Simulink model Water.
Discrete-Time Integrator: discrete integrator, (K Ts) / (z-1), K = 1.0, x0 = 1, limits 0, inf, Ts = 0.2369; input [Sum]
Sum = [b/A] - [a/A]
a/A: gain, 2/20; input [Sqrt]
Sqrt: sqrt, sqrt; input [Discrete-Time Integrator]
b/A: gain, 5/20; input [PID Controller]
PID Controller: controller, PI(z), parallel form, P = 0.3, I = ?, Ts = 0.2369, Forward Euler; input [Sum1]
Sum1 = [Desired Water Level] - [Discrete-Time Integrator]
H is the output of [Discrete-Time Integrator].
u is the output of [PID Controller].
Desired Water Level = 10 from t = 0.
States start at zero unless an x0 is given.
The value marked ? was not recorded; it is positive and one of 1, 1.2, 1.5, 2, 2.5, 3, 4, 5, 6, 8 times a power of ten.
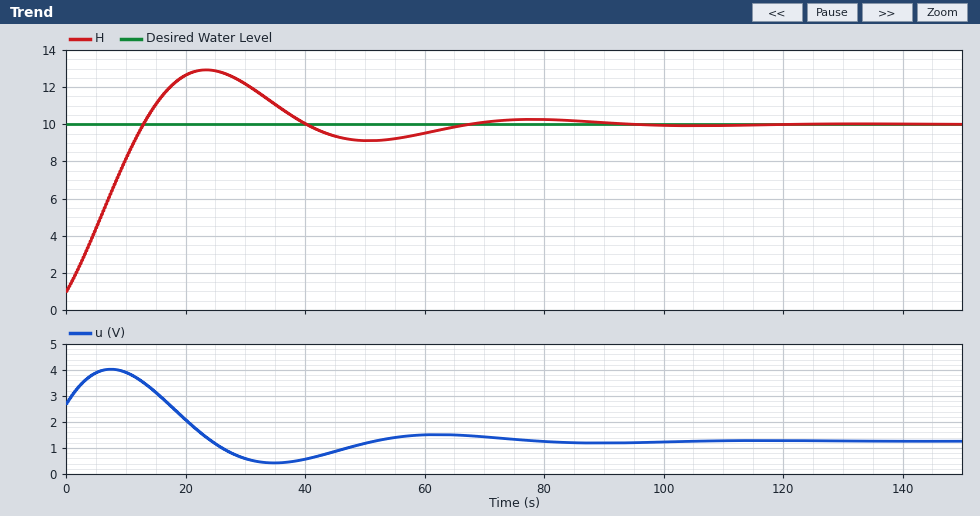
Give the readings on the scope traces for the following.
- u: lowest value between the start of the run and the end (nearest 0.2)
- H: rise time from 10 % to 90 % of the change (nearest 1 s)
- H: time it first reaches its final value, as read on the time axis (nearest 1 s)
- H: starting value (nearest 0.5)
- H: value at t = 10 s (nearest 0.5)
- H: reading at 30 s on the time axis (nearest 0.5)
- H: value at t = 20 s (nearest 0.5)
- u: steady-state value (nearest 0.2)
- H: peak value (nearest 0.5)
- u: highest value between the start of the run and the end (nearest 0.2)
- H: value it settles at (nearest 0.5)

0.4
10 s
13 s
1.0
8.0
12.0
12.5
1.2
13.0
4.0
10.0
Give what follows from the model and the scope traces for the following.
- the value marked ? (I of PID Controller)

0.06
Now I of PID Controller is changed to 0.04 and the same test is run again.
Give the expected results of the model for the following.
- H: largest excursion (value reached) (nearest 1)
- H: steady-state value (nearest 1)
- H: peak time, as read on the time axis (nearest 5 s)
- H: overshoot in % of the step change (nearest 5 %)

12
10
30 s
25 %
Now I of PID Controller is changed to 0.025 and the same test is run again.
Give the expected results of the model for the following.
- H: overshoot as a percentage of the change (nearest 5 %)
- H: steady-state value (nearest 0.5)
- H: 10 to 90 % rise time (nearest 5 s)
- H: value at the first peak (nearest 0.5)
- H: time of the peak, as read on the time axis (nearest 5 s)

15 %
10.0
15 s
11.5
35 s
